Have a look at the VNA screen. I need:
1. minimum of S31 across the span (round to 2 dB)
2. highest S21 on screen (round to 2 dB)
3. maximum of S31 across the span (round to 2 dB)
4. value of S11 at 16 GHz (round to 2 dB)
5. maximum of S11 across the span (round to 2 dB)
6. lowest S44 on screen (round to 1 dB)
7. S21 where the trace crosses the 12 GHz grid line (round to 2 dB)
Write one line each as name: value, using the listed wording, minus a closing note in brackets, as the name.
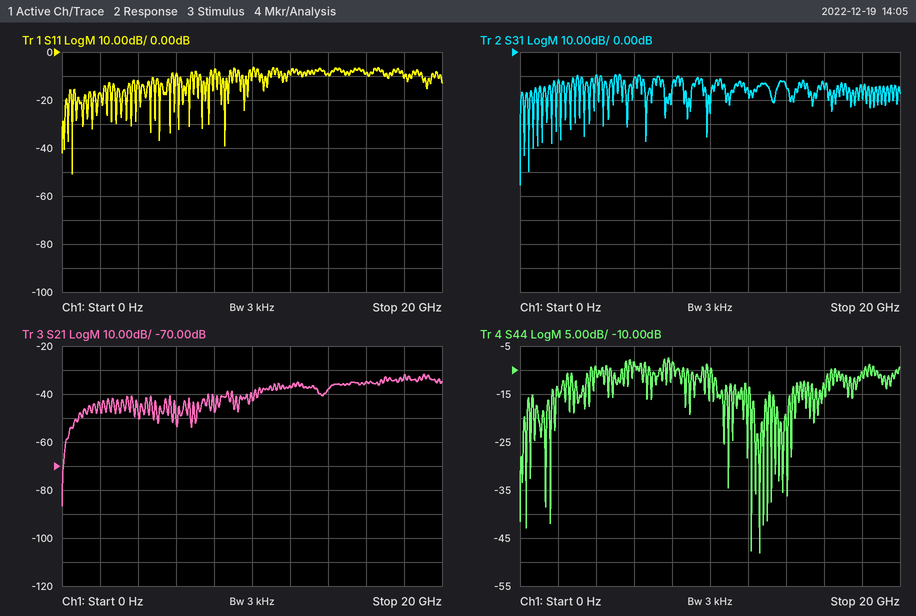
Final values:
minimum of S31 across the span: -56 dB
highest S21 on screen: -32 dB
maximum of S31 across the span: -10 dB
value of S11 at 16 GHz: -8 dB
maximum of S11 across the span: -6 dB
lowest S44 on screen: -48 dB
S21 where the trace crosses the 12 GHz grid line: -36 dB
